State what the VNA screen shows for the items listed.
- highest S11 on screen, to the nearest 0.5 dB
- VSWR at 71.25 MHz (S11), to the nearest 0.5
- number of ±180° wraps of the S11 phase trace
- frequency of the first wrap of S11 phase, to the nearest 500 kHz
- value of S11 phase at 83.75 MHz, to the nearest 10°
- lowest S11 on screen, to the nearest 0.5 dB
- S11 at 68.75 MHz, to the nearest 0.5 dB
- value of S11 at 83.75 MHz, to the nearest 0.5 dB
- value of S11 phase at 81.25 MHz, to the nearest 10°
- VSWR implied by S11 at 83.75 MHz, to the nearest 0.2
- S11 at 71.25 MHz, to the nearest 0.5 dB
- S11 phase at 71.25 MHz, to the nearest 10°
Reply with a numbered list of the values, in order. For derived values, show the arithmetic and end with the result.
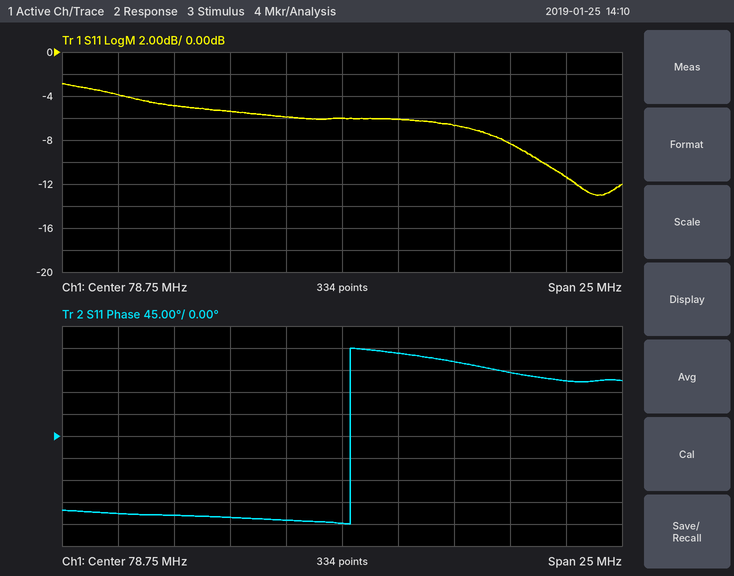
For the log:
1. -3.0 dB
2. |Γ| = 10^(-5/20) = 0.5623; VSWR = (1 + 0.5623)/(1 − 0.5623) ≈ 3.57, so 3.5 to the nearest 0.5
3. 1
4. 79.0 MHz
5. 150°
6. -13.0 dB
7. -4.0 dB
8. -6.5 dB
9. 170°
10. |Γ| = 10^(-6.5/20) = 0.4732; VSWR = (1 + 0.4732)/(1 − 0.4732) ≈ 2.8
11. -5.0 dB
12. -160°
